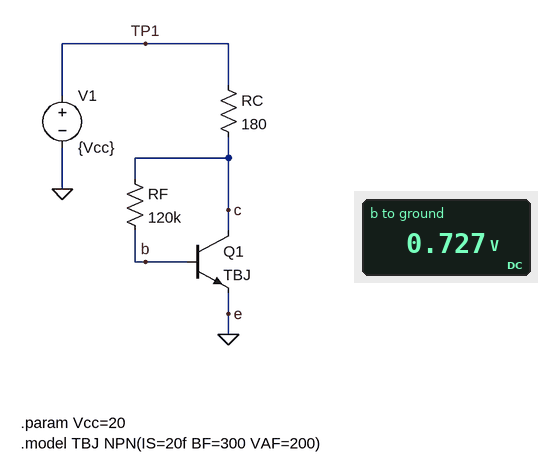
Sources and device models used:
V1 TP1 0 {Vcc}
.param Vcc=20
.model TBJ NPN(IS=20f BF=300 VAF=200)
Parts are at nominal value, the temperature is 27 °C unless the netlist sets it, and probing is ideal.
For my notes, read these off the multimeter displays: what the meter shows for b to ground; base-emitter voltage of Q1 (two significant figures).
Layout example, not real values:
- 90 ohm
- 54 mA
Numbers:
- 0.727 V
- 730 mV
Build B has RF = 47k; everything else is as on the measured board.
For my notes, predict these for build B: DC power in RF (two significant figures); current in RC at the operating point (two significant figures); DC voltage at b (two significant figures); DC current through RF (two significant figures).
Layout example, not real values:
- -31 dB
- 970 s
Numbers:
- 1.6 mW
- 58 mA
- 740 mV
- 190 µA
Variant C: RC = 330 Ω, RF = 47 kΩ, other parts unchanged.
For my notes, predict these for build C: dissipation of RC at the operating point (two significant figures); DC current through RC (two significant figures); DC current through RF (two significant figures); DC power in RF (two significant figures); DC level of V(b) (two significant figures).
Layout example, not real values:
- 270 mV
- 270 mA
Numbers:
- 530 mW
- 40 mA
- 130 µA
- 780 µW
- 730 mV
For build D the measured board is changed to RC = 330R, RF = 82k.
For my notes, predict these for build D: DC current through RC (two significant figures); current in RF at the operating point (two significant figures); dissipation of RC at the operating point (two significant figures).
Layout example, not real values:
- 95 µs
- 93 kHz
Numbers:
- 33 mA
- 100 µA
- 350 mW
